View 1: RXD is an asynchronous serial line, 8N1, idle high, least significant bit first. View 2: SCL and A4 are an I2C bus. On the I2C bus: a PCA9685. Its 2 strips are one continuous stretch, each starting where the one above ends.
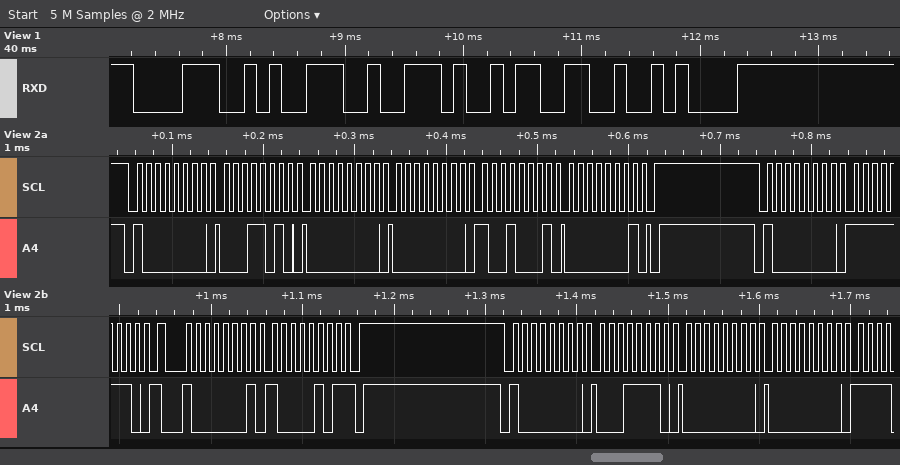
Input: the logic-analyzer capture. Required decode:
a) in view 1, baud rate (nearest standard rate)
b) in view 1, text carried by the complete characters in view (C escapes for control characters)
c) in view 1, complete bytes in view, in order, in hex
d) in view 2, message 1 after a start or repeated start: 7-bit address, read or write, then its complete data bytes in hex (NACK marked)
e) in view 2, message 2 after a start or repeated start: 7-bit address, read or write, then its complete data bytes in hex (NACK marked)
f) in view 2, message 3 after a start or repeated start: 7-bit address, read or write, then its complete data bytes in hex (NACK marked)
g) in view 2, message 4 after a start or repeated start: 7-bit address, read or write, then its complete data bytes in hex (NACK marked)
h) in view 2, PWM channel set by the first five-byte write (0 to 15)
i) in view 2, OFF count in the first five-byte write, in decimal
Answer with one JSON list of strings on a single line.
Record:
["9600 baud", "\"89.3\\n\"", "38 39 2E 33 0A", "0x40 write: 1A 00 00 91 01", "0x40 write: FE", "0x40 read: 85 NACK", "0x40 write: 1E 00 00", "5", "401"]
